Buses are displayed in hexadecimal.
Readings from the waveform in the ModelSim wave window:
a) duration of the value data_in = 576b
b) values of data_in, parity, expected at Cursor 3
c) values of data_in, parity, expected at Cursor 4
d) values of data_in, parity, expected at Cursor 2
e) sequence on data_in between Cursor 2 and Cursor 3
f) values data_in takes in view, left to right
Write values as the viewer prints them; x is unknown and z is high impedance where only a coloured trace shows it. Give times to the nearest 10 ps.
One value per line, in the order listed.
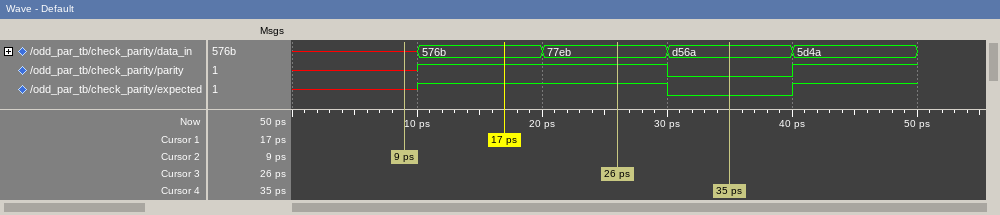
10 ps
data_in=77eb, parity=1, expected=1
data_in=d56a, parity=0, expected=0
data_in=x, parity=x, expected=x
x, 576b, 77eb
x, 576b, 77eb, d56a, 5d4a
